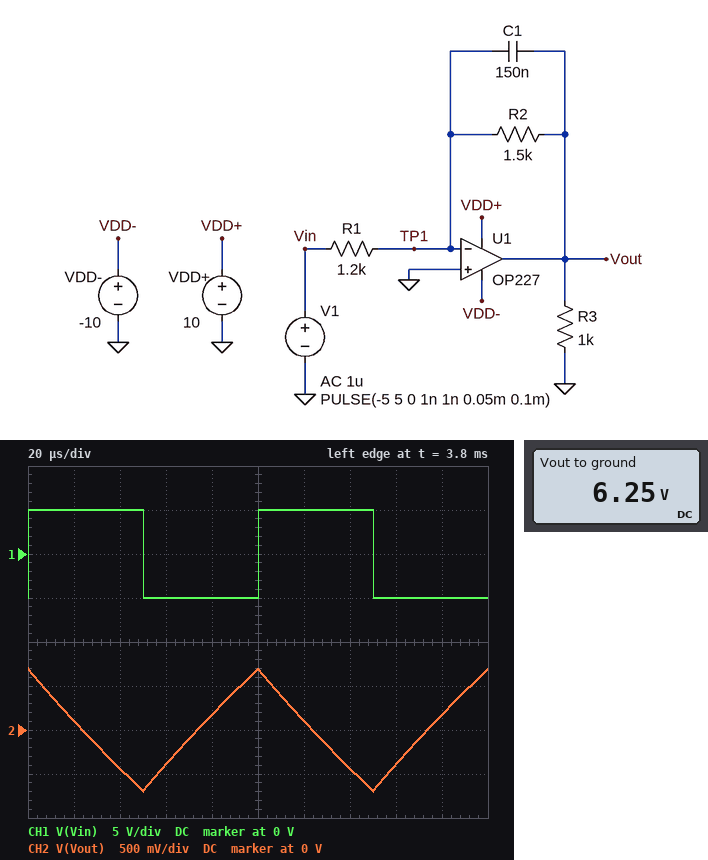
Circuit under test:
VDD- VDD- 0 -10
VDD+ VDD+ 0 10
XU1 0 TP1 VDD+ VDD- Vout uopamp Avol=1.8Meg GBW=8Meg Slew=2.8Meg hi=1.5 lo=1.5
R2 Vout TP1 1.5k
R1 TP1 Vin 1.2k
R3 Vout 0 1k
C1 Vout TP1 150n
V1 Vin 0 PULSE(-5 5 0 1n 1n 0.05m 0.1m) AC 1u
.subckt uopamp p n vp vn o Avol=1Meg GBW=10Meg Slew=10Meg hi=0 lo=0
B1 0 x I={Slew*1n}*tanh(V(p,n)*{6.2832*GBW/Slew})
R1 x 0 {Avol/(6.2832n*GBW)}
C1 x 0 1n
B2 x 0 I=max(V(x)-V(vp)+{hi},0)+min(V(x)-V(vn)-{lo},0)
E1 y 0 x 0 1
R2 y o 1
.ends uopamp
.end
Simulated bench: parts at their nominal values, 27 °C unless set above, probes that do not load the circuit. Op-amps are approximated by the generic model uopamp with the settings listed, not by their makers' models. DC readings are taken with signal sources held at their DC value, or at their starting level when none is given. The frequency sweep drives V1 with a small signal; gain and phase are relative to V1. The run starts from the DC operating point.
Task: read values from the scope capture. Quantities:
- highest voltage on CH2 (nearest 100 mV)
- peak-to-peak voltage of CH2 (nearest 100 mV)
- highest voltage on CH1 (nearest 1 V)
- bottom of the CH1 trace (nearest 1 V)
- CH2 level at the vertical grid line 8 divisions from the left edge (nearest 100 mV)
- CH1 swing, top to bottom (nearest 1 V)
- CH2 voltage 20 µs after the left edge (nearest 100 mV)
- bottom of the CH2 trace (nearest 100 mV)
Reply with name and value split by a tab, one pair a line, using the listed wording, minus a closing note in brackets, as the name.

highest voltage on CH2	700 mV
peak-to-peak voltage of CH2	1.4 V
highest voltage on CH1	5 V
bottom of the CH1 trace	-5 V
CH2 level at the vertical grid line 8 divisions from the left edge	-400 mV
CH1 swing, top to bottom	10 V
CH2 voltage 20 µs after the left edge	100 mV
bottom of the CH2 trace	-700 mV
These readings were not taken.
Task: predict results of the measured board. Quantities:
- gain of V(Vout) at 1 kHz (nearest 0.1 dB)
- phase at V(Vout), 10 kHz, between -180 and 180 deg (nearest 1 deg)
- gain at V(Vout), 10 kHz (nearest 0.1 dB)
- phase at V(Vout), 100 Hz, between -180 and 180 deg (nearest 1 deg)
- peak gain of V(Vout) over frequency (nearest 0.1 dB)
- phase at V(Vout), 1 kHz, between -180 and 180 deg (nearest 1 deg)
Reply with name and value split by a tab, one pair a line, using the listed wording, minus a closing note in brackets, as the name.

gain of V(Vout) at 1 kHz	-2.8 dB
phase at V(Vout), 10 kHz, between -180 and 180 deg	94 deg
gain at V(Vout), 10 kHz	-21.1 dB
phase at V(Vout), 100 Hz, between -180 and 180 deg	172 deg
peak gain of V(Vout) over frequency	1.9 dB
phase at V(Vout), 1 kHz, between -180 and 180 deg	125 deg
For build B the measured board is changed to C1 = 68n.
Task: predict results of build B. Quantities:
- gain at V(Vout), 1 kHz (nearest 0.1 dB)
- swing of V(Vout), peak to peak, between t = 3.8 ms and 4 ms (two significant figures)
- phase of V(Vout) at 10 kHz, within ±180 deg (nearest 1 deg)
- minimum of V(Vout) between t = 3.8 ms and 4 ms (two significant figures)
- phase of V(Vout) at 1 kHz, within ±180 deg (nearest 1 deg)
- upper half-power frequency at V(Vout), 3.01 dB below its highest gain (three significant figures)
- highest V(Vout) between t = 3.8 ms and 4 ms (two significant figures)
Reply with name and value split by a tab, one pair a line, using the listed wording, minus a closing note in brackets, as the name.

gain at V(Vout), 1 kHz	0.4 dB
swing of V(Vout), peak to peak, between t = 3.8 ms and 4 ms	3.0 V
phase of V(Vout) at 10 kHz, within ±180 deg	99 deg
minimum of V(Vout) between t = 3.8 ms and 4 ms	-1.5 V
phase of V(Vout) at 1 kHz, within ±180 deg	147 deg
upper half-power frequency at V(Vout), 3.01 dB below its highest gain	1.56 kHz
highest V(Vout) between t = 3.8 ms and 4 ms	1.5 V
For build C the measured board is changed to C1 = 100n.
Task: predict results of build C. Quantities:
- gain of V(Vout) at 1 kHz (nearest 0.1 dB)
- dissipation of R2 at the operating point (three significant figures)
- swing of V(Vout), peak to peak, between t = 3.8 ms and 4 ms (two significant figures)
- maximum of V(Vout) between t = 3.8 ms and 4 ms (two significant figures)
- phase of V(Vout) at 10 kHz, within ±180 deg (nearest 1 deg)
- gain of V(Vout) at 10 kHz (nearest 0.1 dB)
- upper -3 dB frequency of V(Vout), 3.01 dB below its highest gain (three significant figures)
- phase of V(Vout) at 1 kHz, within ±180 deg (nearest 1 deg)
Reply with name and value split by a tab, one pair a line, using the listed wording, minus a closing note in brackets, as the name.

gain of V(Vout) at 1 kHz	-0.8 dB
dissipation of R2 at the operating point	26.0 mW
swing of V(Vout), peak to peak, between t = 3.8 ms and 4 ms	2.1 V
maximum of V(Vout) between t = 3.8 ms and 4 ms	1.0 V
phase of V(Vout) at 10 kHz, within ±180 deg	96 deg
gain of V(Vout) at 10 kHz	-17.6 dB
upper -3 dB frequency of V(Vout), 3.01 dB below its highest gain	1.06 kHz
phase of V(Vout) at 1 kHz, within ±180 deg	137 deg
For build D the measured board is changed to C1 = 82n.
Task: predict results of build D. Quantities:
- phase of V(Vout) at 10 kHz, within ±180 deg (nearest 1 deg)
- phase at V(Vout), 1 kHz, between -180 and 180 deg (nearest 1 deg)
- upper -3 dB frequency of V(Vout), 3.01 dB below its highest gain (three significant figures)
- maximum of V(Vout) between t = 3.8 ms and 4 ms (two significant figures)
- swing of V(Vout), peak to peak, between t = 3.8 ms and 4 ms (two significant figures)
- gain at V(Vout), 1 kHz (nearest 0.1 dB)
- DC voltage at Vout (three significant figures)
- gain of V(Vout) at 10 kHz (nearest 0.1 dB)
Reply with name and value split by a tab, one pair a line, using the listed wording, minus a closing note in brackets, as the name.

phase of V(Vout) at 10 kHz, within ±180 deg	97 deg
phase at V(Vout), 1 kHz, between -180 and 180 deg	142 deg
upper -3 dB frequency of V(Vout), 3.01 dB below its highest gain	1.29 kHz
maximum of V(Vout) between t = 3.8 ms and 4 ms	1.3 V
swing of V(Vout), peak to peak, between t = 3.8 ms and 4 ms	2.5 V
gain at V(Vout), 1 kHz	-0.1 dB
DC voltage at Vout	6.25 V
gain of V(Vout) at 10 kHz	-15.9 dB
